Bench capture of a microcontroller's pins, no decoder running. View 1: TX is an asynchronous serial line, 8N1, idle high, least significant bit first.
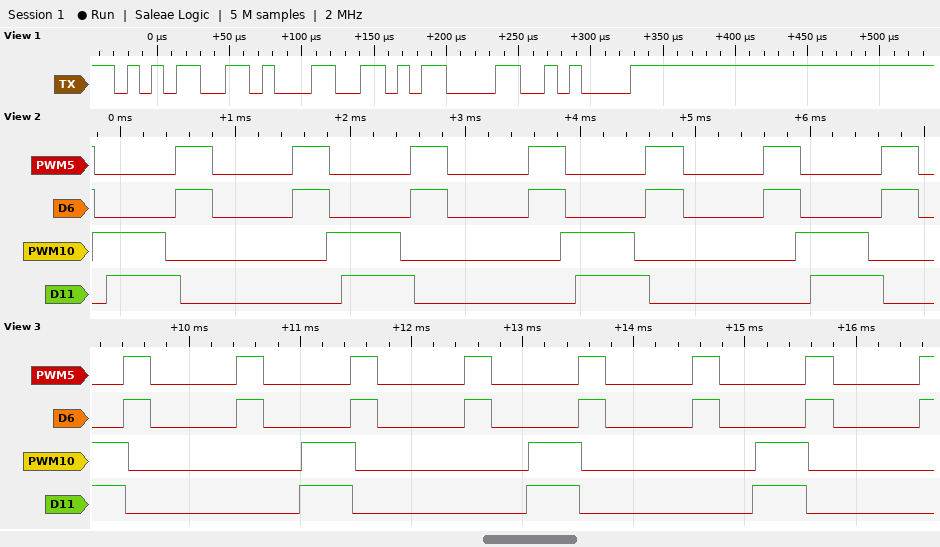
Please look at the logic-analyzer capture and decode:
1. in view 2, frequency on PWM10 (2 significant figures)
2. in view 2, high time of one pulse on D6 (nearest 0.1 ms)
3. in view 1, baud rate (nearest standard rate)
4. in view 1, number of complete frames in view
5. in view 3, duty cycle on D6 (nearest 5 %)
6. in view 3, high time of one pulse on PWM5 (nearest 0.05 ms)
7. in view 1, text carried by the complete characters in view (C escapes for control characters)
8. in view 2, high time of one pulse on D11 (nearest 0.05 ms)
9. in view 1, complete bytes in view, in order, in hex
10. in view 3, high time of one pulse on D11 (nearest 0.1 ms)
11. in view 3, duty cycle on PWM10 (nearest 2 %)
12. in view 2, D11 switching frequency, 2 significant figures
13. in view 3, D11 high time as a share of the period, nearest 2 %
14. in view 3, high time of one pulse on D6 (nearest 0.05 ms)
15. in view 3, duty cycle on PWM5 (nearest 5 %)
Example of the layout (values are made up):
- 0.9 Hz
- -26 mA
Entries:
- 490 Hz
- 0.3 ms
- 115200 baud
- 4
- 25 %
- 0.25 ms
- "51\r\n"
- 0.65 ms
- 35 31 0D 0A
- 0.5 ms
- 24 %
- 490 Hz
- 24 %
- 0.25 ms
- 25 %
